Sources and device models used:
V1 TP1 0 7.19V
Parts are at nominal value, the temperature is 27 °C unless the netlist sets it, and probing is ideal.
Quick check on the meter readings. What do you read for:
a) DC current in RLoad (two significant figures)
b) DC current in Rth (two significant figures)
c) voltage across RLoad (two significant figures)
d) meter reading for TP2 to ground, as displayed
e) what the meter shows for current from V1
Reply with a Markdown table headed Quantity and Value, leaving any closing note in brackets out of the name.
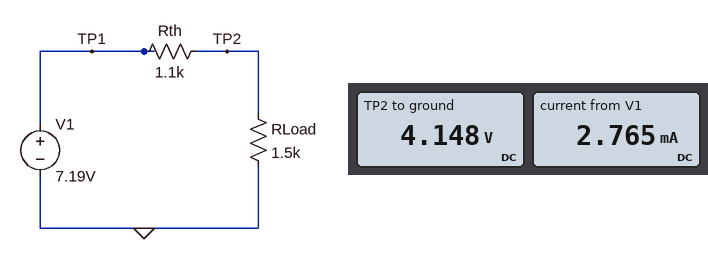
| Quantity | Value |
|---|---|
| DC current in RLoad | 2.8 mA |
| DC current in Rth | 2.8 mA |
| voltage across RLoad | 4.1 V |
| meter reading for TP2 to ground, as displayed | 4.148 V |
| what the meter shows for current from V1 | 2.765 mA |
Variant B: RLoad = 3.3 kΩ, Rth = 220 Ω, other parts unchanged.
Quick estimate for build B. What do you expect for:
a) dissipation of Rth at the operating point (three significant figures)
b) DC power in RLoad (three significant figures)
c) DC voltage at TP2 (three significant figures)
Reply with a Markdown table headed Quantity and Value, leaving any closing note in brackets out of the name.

| Quantity | Value |
|---|---|
| dissipation of Rth at the operating point | 918 µW |
| DC power in RLoad | 13.8 mW |
| DC voltage at TP2 | 6.74 V |
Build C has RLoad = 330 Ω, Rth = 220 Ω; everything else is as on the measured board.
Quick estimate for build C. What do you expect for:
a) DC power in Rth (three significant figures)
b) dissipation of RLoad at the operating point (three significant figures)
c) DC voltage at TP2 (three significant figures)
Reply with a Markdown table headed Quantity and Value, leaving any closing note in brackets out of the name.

| Quantity | Value |
|---|---|
| DC power in Rth | 37.6 mW |
| dissipation of RLoad at the operating point | 56.4 mW |
| DC voltage at TP2 | 4.31 V |
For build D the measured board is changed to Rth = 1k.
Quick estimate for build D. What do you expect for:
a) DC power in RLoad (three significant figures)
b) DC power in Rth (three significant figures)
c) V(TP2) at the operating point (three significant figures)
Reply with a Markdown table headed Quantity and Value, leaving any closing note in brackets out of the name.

| Quantity | Value |
|---|---|
| DC power in RLoad | 12.4 mW |
| DC power in Rth | 8.27 mW |
| V(TP2) at the operating point | 4.31 V |
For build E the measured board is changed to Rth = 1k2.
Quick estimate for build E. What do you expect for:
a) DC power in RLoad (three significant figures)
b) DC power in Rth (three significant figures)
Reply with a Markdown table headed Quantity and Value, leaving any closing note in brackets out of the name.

| Quantity | Value |
|---|---|
| DC power in RLoad | 10.6 mW |
| DC power in Rth | 8.51 mW |
